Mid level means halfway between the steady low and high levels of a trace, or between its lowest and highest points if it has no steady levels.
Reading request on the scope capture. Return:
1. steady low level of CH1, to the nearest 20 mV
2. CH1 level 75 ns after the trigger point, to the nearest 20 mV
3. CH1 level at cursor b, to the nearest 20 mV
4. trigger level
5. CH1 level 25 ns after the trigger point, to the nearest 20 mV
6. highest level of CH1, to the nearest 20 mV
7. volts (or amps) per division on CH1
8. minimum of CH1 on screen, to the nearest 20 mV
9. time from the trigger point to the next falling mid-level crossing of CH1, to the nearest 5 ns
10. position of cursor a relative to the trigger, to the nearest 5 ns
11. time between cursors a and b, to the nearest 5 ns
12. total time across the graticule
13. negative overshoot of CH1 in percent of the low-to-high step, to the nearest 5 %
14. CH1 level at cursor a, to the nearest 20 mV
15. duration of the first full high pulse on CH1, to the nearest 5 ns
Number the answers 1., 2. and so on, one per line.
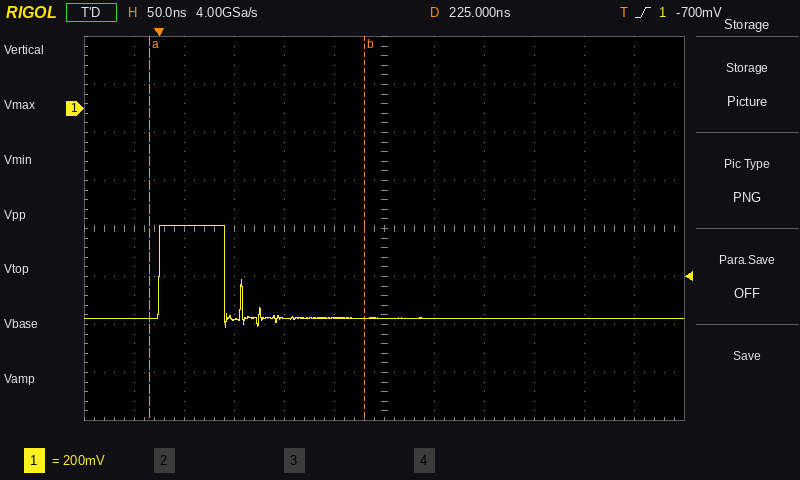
1. -880 mV
2. -880 mV
3. -880 mV
4. -700 mV
5. -480 mV
6. -480 mV
7. 200 mV
8. -920 mV
9. 65 ns
10. -10 ns
11. 215 ns
12. 600 ns
13. 10 %
14. -880 mV
15. 65 ns
